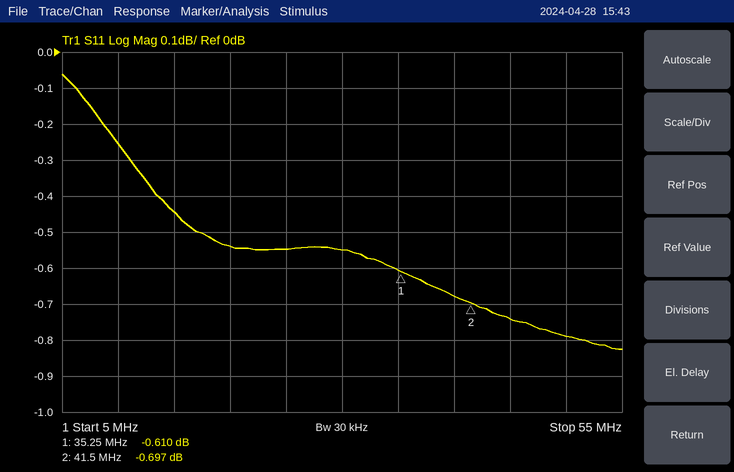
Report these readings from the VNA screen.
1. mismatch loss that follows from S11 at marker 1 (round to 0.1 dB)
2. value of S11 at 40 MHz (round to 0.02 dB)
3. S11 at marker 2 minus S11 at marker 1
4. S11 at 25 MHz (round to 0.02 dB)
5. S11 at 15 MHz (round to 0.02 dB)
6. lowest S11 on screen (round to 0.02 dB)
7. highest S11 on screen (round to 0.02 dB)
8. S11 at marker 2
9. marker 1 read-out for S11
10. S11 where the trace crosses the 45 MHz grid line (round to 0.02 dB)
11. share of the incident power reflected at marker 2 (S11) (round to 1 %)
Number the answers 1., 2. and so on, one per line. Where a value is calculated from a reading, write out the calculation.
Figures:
1. −10 log10(1 − 10^(-0.61/10)) ≈ 8.8 dB
2. -0.68 dB
3. -0.697 − (-0.61) = -0.087 dB
4. -0.54 dB
5. -0.44 dB
6. -0.82 dB
7. -0.06 dB
8. -0.697 dB
9. -0.610 dB
10. -0.74 dB
11. 10^(-0.697/10) ≈ 85 %
